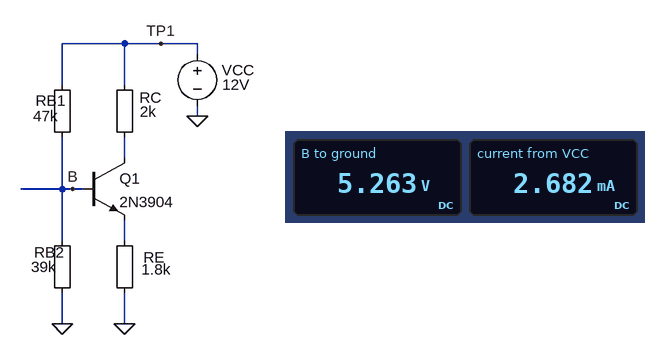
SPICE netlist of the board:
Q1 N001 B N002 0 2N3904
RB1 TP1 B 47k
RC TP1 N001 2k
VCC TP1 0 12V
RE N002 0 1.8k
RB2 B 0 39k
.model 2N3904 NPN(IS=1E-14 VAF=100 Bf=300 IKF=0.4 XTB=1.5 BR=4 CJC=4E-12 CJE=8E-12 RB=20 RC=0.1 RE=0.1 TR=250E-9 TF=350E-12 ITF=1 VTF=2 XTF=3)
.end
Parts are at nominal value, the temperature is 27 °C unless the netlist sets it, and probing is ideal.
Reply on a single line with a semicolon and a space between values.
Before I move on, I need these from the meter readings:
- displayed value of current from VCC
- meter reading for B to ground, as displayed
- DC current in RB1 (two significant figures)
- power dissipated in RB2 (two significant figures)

2.682 mA; 5.263 V; 140 µA; 710 µW
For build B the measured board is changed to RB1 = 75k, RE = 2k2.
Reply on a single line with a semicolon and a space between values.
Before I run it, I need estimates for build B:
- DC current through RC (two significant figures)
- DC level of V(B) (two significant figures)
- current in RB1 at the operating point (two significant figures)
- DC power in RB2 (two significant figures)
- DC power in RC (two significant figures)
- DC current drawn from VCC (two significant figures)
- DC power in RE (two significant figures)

1.5 mA; 4.0 V; 110 µA; 410 µW; 4.5 mW; 1.6 mA; 5.0 mW
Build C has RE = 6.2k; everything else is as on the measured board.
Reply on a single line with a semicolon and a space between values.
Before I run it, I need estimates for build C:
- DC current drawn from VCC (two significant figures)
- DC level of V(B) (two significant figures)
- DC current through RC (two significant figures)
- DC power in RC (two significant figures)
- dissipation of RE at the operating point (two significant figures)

900 µA; 5.4 V; 760 µA; 1.2 mW; 3.6 mW
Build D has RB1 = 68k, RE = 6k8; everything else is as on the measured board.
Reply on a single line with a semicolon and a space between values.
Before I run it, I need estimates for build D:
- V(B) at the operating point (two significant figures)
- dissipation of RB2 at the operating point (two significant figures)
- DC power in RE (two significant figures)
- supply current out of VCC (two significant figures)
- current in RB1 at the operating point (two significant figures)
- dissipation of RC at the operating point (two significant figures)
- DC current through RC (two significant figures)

4.3 V; 480 µW; 2.0 mW; 650 µA; 110 µA; 590 µW; 540 µA
